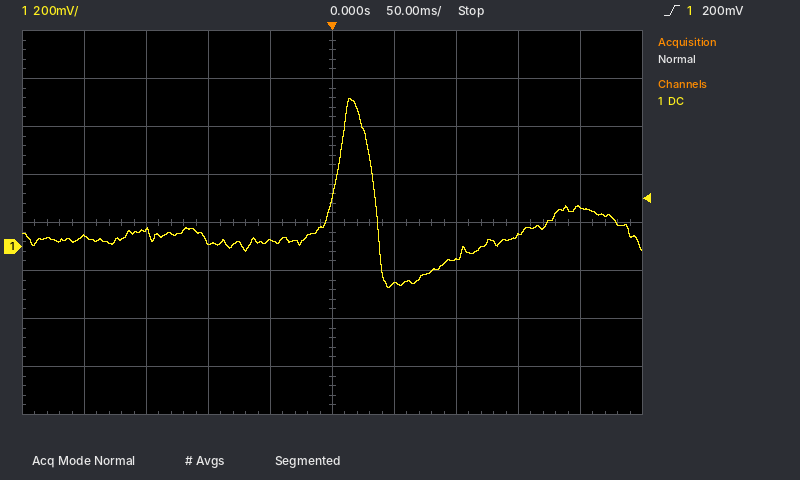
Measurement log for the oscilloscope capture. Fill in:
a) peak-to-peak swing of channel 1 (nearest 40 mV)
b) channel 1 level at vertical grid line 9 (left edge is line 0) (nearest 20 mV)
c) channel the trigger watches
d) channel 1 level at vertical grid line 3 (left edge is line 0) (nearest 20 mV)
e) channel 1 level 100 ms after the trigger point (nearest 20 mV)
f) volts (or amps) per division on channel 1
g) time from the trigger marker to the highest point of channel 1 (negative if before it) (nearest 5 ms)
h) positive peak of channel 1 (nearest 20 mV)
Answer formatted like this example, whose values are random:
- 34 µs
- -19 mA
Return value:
- 800 mV
- 160 mV
- channel 1
- 20 mV
- -60 mV
- 200 mV
- +15 ms
- 620 mV
